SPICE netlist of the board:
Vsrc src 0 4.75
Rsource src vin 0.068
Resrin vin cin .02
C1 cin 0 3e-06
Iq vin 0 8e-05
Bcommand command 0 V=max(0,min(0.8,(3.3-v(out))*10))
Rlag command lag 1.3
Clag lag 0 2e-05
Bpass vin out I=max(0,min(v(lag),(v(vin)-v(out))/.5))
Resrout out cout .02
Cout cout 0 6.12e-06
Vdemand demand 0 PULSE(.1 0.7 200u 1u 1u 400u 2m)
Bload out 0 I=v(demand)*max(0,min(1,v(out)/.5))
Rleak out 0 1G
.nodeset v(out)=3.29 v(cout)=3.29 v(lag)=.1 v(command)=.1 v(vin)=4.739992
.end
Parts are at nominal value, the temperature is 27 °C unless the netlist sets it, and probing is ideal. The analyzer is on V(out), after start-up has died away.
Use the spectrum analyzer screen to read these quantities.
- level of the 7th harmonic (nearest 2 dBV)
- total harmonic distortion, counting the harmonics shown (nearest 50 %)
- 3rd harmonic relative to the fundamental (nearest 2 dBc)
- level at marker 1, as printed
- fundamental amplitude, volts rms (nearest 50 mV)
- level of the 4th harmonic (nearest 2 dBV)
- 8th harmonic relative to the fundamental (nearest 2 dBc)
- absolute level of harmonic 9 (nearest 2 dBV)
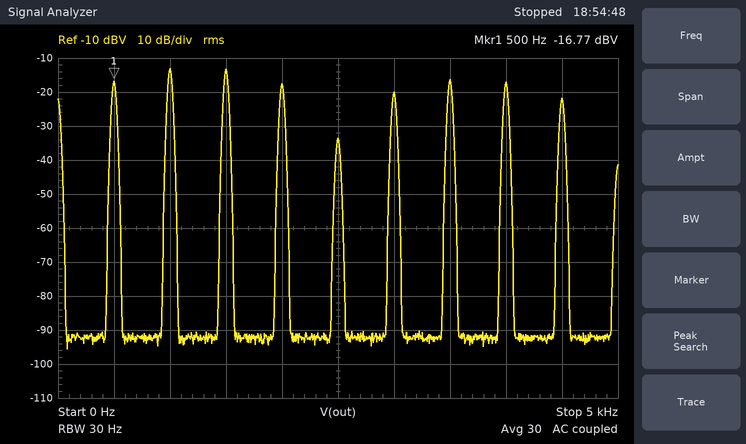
-16 dBV
300 %
4 dBc
-16.77 dBV
150 mV
-18 dBV
0 dBc
-22 dBV
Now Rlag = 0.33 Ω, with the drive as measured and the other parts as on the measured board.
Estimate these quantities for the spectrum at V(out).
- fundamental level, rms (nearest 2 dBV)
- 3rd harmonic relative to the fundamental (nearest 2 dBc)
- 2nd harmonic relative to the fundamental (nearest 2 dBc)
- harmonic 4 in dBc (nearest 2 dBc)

-34 dBV
0 dBc
0 dBc
-6 dBc
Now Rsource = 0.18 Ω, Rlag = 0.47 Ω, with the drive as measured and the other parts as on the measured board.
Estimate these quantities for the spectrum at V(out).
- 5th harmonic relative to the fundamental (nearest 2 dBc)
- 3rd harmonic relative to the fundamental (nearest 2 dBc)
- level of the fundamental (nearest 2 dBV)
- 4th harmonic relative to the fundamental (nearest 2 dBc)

-40 dBc
2 dBc
-32 dBV
-2 dBc
